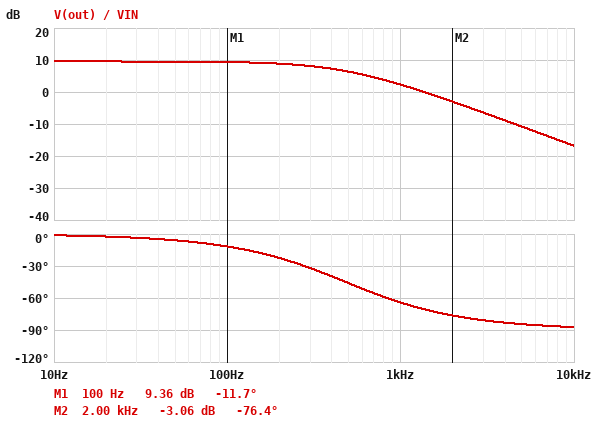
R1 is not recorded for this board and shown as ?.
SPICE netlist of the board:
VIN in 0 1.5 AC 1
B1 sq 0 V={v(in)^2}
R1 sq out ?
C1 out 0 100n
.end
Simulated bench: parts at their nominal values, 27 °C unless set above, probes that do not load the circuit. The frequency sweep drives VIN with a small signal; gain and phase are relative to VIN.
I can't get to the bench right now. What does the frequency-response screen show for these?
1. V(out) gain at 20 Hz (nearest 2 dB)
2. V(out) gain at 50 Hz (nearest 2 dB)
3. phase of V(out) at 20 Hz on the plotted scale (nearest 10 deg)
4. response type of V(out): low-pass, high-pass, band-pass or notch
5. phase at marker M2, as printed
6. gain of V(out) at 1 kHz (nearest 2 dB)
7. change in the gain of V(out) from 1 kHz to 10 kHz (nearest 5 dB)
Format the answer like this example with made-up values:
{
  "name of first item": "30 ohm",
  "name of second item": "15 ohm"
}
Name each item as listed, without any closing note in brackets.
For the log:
{
  "V(out) gain at 20 Hz": "10 dB",
  "V(out) gain at 50 Hz": "10 dB",
  "phase of V(out) at 20 Hz on the plotted scale": "0 deg",
  "response type of V(out): low-pass, high-pass, band-pass or notch": "low-pass",
  "phase at marker M2, as printed": "-76.4 deg",
  "gain of V(out) at 1 kHz": "2 dB",
  "change in the gain of V(out) from 1 kHz to 10 kHz": "-20 dB"
}
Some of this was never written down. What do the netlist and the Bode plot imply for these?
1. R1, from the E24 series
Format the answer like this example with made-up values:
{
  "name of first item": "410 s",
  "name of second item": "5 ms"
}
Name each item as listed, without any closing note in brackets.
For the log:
{
  "R1, from the E24 series": "3.3 kΩ"
}
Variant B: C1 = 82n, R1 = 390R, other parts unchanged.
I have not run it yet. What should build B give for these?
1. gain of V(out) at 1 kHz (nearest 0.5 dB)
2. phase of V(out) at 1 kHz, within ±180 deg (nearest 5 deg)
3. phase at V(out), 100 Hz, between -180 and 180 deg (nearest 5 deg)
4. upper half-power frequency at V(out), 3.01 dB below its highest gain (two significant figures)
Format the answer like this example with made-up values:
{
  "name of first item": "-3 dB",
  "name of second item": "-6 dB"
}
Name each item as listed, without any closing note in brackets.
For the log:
{
  "gain of V(out) at 1 kHz": "9.5 dB",
  "phase of V(out) at 1 kHz, within ±180 deg": "-10 deg",
  "phase at V(out), 100 Hz, between -180 and 180 deg": "0 deg",
  "upper half-power frequency at V(out), 3.01 dB below its highest gain": "5.0 kHz"
}
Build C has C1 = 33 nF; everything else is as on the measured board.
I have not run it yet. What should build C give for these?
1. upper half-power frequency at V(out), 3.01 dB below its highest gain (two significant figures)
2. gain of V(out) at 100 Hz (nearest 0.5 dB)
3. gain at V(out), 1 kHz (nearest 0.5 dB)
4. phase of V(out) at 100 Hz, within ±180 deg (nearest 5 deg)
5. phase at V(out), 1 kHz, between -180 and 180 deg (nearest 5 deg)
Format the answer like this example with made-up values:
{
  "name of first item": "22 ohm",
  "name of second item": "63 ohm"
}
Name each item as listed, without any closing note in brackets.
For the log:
{
  "upper half-power frequency at V(out), 3.01 dB below its highest gain": "1.5 kHz",
  "gain of V(out) at 100 Hz": "9.5 dB",
  "gain at V(out), 1 kHz": "8.0 dB",
  "phase of V(out) at 100 Hz, within ±180 deg": "-5 deg",
  "phase at V(out), 1 kHz, between -180 and 180 deg": "-35 deg"
}
